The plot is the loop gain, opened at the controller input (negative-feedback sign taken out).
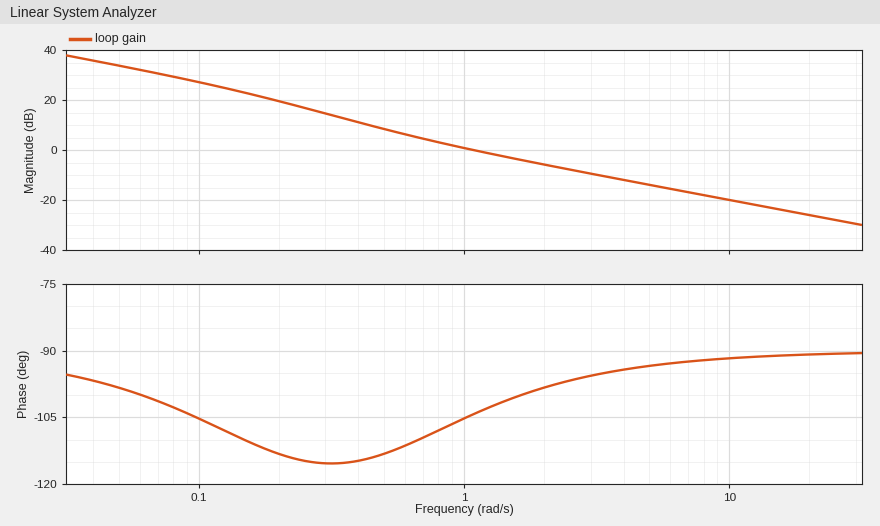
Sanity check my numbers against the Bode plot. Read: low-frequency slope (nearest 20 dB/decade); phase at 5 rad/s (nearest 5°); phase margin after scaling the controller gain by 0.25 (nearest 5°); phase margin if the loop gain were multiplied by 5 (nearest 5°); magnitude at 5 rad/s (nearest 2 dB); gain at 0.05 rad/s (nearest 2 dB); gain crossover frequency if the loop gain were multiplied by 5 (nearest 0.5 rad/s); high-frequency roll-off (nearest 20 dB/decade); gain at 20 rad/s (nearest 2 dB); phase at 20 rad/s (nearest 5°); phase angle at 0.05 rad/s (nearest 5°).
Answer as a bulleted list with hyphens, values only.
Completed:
- -20 dB/decade
- -95°
- 65°
- 85°
- -14 dB
- 34 dB
- 5.0 rad/s
- -20 dB/decade
- -26 dB
- -90°
- -100°
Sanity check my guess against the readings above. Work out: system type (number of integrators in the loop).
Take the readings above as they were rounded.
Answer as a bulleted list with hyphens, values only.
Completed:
- 1
